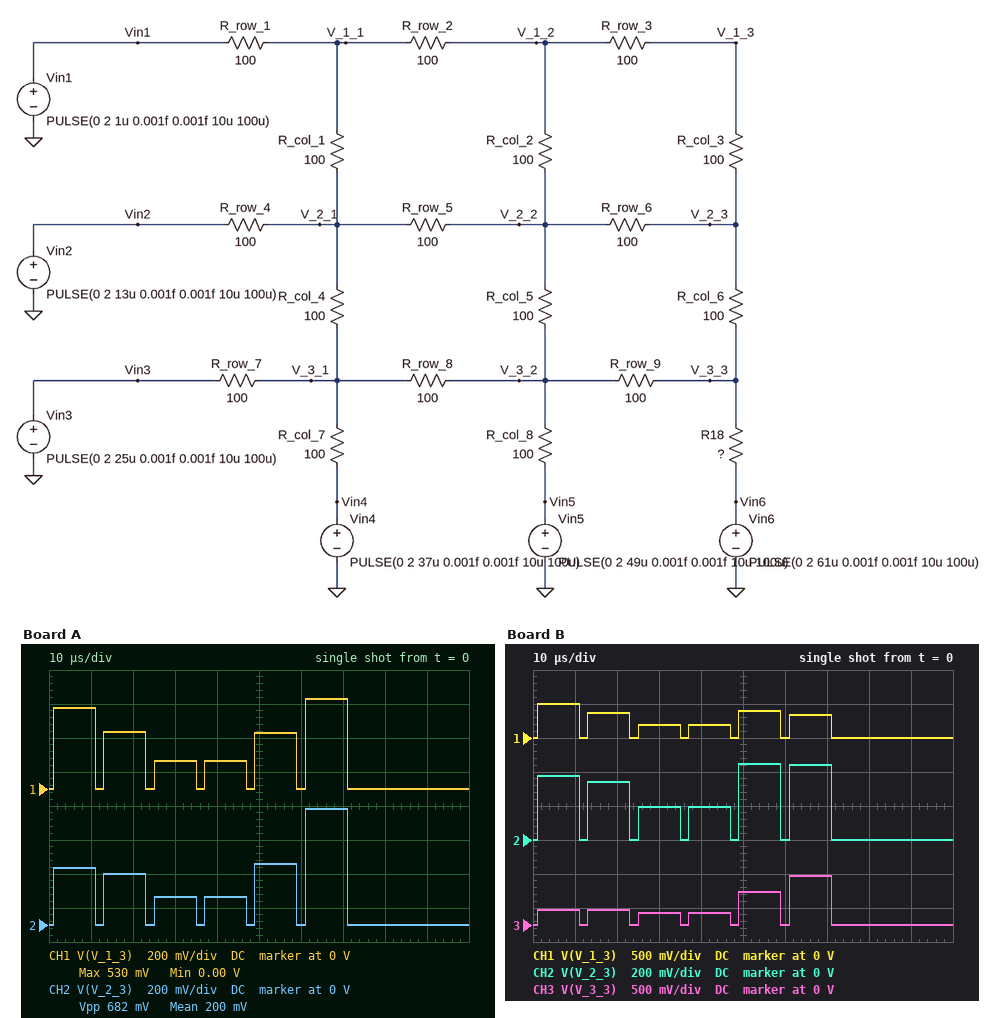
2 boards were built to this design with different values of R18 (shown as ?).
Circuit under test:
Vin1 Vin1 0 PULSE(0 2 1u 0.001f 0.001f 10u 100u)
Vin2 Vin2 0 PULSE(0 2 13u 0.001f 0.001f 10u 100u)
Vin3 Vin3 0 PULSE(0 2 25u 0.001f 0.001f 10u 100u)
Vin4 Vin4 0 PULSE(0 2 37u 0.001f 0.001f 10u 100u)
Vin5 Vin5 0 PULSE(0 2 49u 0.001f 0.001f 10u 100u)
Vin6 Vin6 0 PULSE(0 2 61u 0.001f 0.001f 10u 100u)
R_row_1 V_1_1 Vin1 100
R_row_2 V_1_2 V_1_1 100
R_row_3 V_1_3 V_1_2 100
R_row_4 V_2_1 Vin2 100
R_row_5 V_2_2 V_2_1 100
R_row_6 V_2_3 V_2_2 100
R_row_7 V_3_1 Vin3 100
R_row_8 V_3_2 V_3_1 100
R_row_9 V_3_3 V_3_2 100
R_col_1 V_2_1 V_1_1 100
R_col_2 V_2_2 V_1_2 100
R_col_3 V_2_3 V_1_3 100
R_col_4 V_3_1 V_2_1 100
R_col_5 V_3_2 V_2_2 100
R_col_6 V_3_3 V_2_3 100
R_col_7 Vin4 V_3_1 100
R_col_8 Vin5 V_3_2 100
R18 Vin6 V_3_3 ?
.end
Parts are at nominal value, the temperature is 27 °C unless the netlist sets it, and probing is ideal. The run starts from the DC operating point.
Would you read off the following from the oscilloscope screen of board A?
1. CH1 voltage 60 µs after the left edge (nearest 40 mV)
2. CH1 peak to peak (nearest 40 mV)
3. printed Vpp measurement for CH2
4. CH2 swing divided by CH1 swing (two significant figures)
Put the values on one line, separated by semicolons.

0 V; 520 mV; 682 mV; 1.3
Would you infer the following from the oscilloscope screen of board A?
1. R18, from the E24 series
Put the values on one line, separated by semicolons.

82 Ω
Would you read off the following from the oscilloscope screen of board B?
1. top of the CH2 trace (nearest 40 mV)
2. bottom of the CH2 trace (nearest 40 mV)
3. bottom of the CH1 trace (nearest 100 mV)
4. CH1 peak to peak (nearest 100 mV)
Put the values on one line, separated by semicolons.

440 mV; 0 V; 0 V; 500 mV
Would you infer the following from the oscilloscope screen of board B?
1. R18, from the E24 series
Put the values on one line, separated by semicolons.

180 Ω
